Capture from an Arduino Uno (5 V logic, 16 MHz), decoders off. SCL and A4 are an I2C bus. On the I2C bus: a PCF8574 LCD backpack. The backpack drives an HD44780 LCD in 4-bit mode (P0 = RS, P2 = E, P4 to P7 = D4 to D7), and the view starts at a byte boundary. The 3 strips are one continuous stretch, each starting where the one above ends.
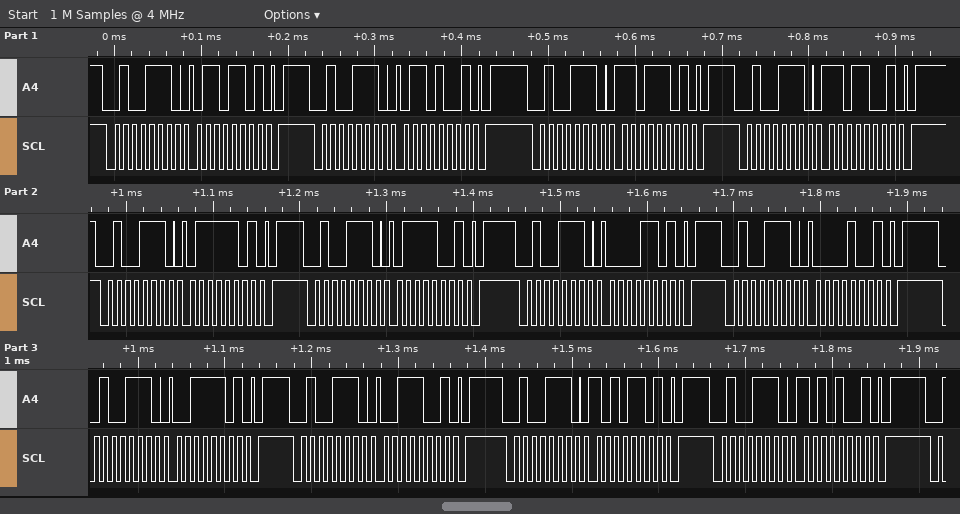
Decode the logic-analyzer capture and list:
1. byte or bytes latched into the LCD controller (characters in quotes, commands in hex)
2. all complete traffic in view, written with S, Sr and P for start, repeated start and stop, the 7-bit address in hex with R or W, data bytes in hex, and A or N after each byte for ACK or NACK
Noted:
'm' 'p' ':'
S 27W A 6D A P S 27W A 69 A P S 27W A DD A P S 27W A D9 A P S 27W A 7D A P S 27W A 79 A P S 27W A 0D A P S 27W A 09 A P S 27W A 3D A P S 27W A 39 A P S 27W A AD A P S 27W A A9 A P
